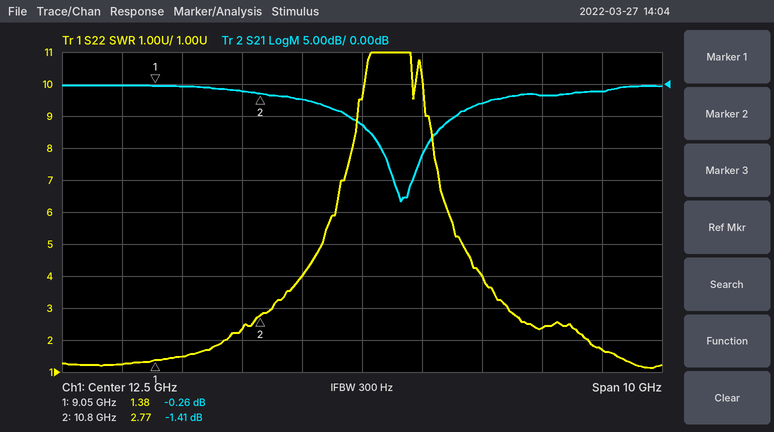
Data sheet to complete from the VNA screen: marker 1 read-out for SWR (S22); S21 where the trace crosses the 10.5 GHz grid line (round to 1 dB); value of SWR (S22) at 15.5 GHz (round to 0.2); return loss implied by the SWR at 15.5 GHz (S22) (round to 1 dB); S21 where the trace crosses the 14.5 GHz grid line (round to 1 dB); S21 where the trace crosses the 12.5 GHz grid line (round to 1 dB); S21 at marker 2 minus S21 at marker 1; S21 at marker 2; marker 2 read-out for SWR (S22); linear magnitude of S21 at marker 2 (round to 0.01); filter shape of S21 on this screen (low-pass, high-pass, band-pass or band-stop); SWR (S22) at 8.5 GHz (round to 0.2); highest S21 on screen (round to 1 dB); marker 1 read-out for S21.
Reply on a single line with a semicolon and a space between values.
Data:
1.38; -1 dB; 2.4; 8 dB; -3 dB; -6 dB; -1.15 dB; -1.41 dB; 2.77; 0.85; band-stop; 1.2; 0 dB; -0.26 dB
